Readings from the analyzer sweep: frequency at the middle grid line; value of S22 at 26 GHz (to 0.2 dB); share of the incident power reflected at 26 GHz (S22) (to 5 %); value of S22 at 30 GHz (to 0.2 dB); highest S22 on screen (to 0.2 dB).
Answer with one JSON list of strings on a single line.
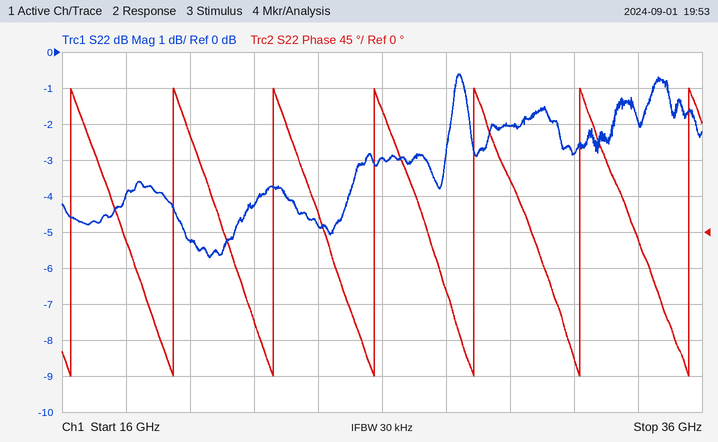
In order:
["26 GHz", "-3.0 dB", "50 %", "-2.0 dB", "-0.6 dB"]
